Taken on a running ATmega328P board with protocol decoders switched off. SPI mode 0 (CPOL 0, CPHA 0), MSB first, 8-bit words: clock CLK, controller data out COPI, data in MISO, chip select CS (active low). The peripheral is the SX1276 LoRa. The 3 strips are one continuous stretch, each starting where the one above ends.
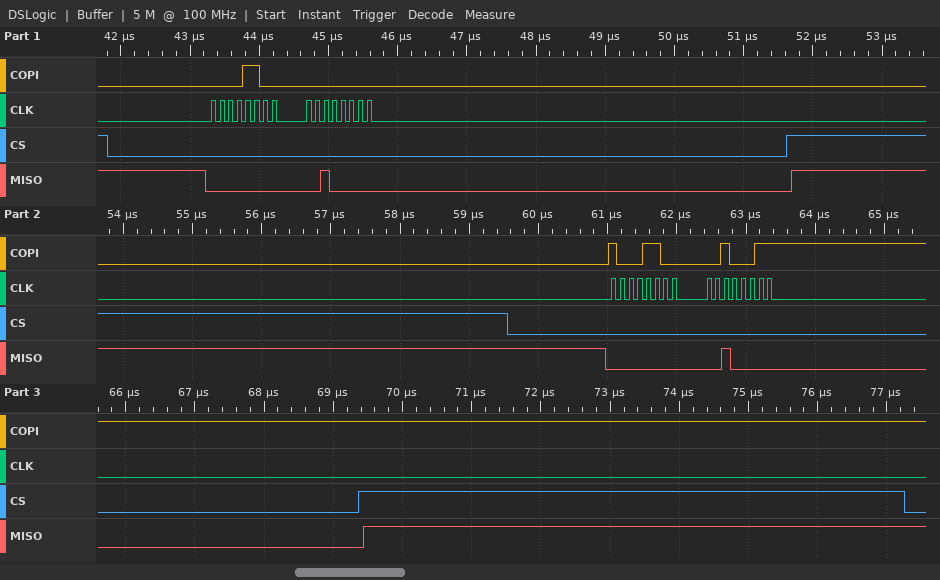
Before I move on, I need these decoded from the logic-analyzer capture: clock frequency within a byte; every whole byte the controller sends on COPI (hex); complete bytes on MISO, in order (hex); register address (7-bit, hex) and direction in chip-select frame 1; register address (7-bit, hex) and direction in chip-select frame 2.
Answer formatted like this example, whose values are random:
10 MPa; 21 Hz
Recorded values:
8 MHz; 0x0C 0x00 0x8C 0x23; 0x00 0x20 0x00 0x20; 0x0C read; 0x0C write
